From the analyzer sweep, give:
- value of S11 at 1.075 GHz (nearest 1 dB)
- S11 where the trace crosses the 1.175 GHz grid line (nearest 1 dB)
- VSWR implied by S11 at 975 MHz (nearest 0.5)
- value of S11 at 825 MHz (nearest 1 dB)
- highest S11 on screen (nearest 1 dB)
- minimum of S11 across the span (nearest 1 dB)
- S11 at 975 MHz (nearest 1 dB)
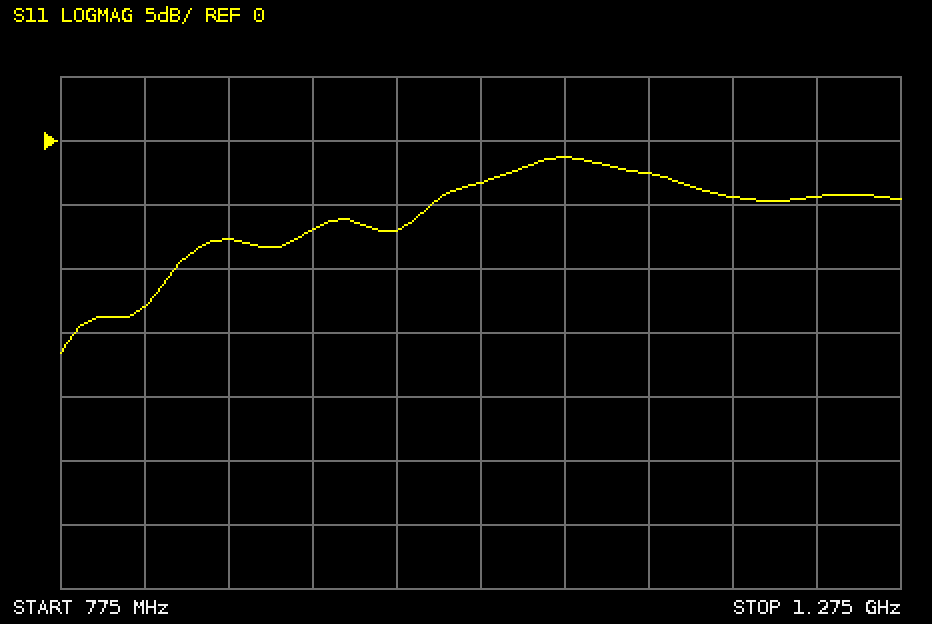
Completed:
-1 dB
-4 dB
2.5
-13 dB
-1 dB
-17 dB
-7 dB
